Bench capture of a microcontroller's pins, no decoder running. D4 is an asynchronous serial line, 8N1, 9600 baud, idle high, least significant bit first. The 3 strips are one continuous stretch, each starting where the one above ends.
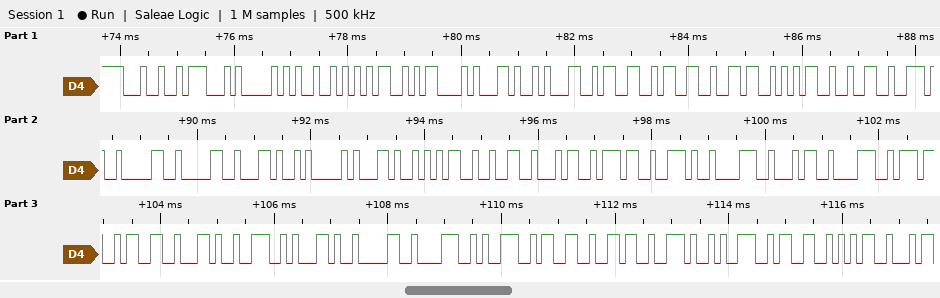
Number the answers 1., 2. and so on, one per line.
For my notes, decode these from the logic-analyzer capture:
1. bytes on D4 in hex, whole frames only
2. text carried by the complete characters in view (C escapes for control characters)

1. 24 47 50 52 4D 43 2C 31 33 33 36 35 32 2E 30 30 2C 41 2C 35 32 34 37 2E 38 34 38 37 33 2C 4E 2C 30 38 39 33 36 2E 39 33 35
2. "$GPRMC,133652.00,A,5247.84873,N,08936.935"
